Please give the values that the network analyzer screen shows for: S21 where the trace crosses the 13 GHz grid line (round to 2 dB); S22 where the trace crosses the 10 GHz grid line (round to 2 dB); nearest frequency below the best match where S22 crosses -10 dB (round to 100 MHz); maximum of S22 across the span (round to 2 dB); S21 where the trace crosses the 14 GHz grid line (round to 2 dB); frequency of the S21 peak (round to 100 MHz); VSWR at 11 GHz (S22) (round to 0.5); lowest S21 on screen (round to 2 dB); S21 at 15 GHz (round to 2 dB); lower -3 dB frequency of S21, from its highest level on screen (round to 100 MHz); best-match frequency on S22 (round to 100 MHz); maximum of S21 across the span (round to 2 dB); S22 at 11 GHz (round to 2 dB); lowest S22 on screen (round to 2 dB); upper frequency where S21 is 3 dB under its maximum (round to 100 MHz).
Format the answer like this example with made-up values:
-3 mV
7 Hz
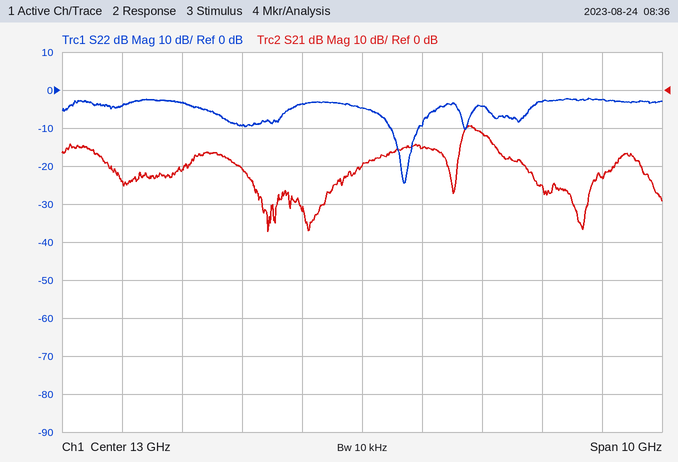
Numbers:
-20 dB
-4 dB
13.5 GHz
-2 dB
-16 dB
14.8 GHz
2.0
-38 dB
-12 dB
14.7 GHz
13.7 GHz
-10 dB
-10 dB
-24 dB
15.1 GHz
